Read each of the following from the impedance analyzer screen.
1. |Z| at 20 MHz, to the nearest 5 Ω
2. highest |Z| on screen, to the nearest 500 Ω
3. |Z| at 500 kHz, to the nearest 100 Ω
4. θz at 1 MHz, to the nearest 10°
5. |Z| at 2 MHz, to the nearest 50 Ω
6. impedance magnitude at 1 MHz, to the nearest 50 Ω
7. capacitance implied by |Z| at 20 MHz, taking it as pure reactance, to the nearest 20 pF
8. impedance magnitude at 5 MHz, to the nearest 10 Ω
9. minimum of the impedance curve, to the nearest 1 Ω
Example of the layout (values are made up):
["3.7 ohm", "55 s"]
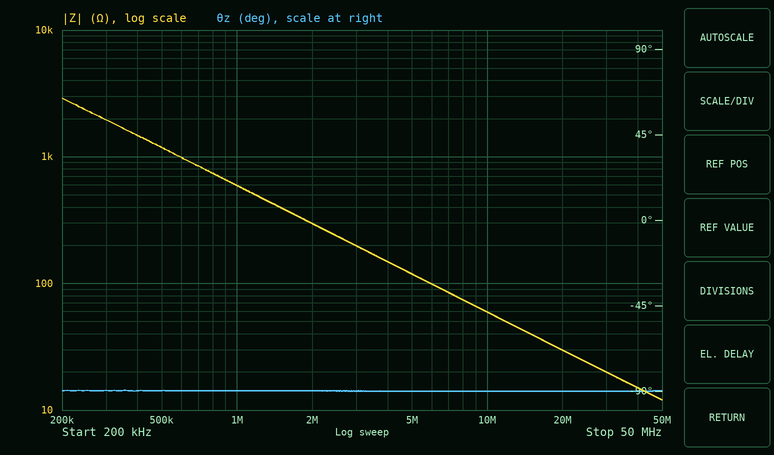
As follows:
["30 Ω", "3.0 kΩ", "1.2 kΩ", "-90°", "300 Ω", "600 Ω", "260 pF", "120 Ω", "12 Ω"]
